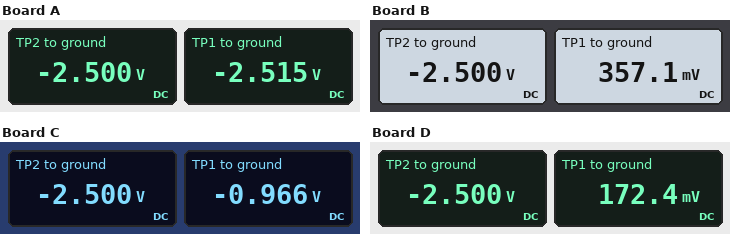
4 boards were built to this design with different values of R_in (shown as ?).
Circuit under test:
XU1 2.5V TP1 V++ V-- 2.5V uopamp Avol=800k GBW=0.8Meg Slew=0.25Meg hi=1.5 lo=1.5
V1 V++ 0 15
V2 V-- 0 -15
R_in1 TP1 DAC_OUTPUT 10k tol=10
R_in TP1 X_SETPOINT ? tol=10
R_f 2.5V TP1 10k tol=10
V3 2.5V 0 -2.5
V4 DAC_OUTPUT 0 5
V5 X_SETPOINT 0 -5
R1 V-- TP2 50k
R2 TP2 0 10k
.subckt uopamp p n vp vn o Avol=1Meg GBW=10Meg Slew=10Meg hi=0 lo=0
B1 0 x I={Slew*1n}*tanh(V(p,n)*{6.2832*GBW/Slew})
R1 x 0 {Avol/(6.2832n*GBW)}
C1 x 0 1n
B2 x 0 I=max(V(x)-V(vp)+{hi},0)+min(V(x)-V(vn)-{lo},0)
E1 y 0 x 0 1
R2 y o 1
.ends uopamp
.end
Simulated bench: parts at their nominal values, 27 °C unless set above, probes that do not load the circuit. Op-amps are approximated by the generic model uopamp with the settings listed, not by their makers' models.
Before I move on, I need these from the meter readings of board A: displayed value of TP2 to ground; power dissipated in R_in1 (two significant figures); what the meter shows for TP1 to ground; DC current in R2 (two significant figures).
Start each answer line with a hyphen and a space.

- -2.500 V
- 5.6 mW
- -2.515 V
- 250 µA
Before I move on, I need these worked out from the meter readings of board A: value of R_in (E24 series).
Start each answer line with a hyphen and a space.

- 3.3 kΩ
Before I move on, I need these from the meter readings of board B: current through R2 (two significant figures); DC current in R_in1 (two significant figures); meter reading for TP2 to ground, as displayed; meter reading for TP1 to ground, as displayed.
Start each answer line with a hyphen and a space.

- 250 µA
- 460 µA
- -2.500 V
- 357.1 mV
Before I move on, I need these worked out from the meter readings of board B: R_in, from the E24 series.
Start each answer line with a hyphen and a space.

- 30 kΩ
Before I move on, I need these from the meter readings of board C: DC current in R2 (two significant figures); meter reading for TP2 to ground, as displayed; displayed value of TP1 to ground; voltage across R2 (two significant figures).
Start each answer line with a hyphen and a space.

- 250 µA
- -2.500 V
- -0.966 V
- 2.5 V
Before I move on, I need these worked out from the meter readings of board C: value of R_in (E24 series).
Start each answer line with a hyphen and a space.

- 9.1 kΩ
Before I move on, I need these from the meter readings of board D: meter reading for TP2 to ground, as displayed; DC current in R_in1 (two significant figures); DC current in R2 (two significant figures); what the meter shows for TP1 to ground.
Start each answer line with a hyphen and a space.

- -2.500 V
- 480 µA
- 250 µA
- 172.4 mV
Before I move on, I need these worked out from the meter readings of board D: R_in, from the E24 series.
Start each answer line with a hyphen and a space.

- 24 kΩ
